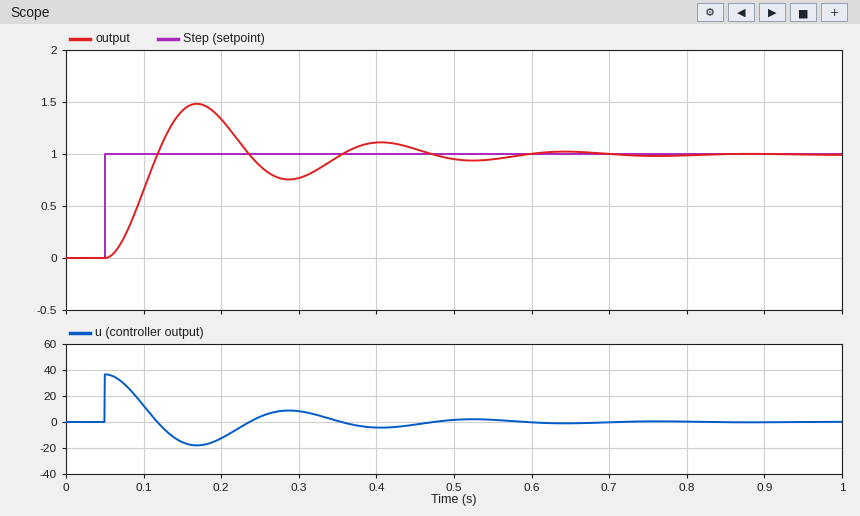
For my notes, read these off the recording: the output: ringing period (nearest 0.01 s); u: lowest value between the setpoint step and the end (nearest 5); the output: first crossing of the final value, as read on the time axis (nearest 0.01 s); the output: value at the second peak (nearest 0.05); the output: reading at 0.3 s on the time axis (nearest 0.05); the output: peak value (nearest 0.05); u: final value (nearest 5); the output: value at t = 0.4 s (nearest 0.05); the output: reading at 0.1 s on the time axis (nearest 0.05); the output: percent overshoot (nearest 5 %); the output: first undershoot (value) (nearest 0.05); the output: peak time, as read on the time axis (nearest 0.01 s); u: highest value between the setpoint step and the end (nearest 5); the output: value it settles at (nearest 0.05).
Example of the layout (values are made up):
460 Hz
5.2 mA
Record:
0.24 s
-20
0.12 s
1.10
0.75
1.50
0
1.10
0.65
50 %
0.75
0.17 s
35
1.00
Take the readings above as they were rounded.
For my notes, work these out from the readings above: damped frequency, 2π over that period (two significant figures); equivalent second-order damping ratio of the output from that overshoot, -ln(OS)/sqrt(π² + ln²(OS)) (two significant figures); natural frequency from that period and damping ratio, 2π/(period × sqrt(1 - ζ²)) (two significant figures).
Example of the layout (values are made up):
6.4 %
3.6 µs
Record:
26 rad/s
0.22
27 rad/s
